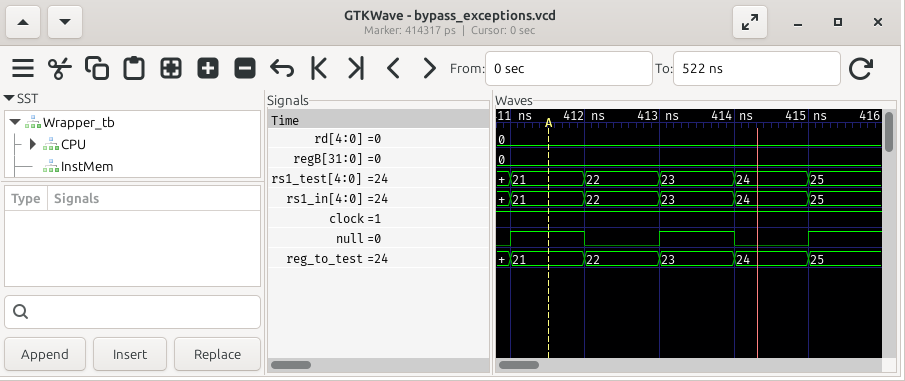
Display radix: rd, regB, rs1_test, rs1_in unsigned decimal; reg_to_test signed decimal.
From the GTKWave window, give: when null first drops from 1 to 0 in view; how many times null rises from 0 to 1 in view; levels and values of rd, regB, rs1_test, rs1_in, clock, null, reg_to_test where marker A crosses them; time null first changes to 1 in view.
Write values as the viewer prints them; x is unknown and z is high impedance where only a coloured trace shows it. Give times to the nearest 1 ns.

412 ns
3
rd=0, regB=0, rs1_test=21, rs1_in=21, clock=1, null=1, reg_to_test=21
411 ns
